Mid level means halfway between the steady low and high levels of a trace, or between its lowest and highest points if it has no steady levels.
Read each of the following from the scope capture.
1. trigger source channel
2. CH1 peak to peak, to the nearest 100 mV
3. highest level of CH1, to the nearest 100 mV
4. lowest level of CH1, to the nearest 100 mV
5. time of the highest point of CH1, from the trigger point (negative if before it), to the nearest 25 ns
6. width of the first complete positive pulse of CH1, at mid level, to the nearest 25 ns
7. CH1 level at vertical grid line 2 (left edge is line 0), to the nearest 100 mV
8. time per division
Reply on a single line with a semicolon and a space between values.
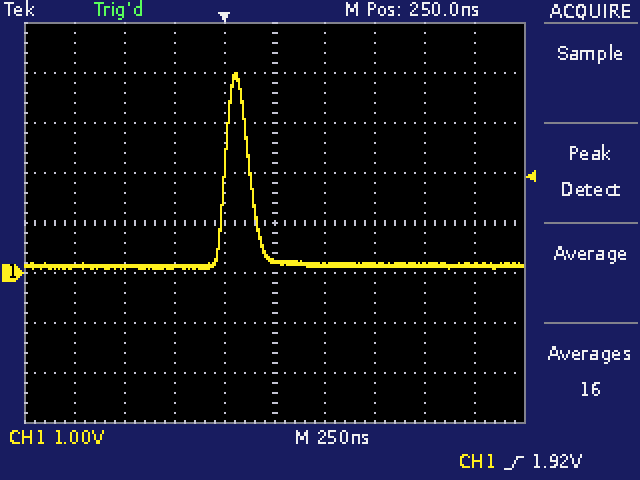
CH1; 3.9 V; 4.0 V; 100 mV; +50 ns; 125 ns; 100 mV; 250 ns
